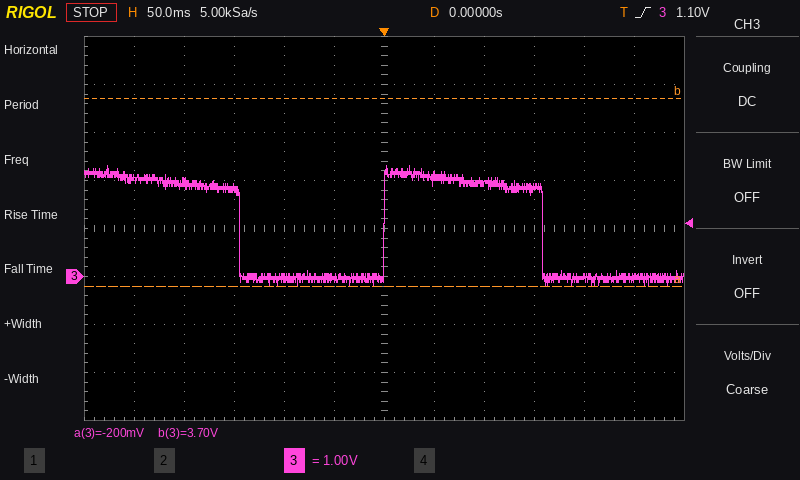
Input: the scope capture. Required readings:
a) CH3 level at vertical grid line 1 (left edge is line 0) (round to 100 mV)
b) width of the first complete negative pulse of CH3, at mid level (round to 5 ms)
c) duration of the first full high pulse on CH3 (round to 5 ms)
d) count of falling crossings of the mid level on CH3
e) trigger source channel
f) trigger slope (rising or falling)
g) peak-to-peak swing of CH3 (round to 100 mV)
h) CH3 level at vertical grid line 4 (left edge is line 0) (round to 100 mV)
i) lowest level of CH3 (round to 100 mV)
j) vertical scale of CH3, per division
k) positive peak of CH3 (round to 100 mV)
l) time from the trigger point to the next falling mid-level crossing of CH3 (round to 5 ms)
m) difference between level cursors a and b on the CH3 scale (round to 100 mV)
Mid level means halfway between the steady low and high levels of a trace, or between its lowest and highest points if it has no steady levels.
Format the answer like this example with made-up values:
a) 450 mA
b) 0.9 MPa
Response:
a) 2.0 V
b) 145 ms
c) 160 ms
d) 2
e) CH3
f) rising
g) 2.5 V
h) 0.0 V
i) -200 mV
j) 1 V
k) 2.3 V
l) 160 ms
m) 3.9 V
